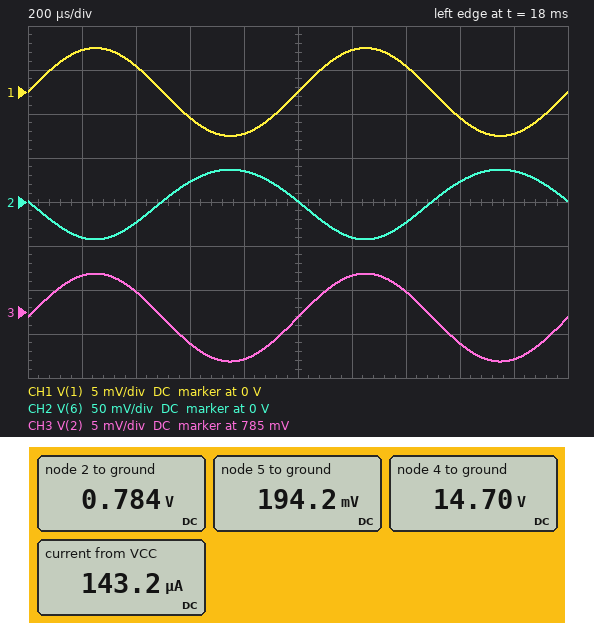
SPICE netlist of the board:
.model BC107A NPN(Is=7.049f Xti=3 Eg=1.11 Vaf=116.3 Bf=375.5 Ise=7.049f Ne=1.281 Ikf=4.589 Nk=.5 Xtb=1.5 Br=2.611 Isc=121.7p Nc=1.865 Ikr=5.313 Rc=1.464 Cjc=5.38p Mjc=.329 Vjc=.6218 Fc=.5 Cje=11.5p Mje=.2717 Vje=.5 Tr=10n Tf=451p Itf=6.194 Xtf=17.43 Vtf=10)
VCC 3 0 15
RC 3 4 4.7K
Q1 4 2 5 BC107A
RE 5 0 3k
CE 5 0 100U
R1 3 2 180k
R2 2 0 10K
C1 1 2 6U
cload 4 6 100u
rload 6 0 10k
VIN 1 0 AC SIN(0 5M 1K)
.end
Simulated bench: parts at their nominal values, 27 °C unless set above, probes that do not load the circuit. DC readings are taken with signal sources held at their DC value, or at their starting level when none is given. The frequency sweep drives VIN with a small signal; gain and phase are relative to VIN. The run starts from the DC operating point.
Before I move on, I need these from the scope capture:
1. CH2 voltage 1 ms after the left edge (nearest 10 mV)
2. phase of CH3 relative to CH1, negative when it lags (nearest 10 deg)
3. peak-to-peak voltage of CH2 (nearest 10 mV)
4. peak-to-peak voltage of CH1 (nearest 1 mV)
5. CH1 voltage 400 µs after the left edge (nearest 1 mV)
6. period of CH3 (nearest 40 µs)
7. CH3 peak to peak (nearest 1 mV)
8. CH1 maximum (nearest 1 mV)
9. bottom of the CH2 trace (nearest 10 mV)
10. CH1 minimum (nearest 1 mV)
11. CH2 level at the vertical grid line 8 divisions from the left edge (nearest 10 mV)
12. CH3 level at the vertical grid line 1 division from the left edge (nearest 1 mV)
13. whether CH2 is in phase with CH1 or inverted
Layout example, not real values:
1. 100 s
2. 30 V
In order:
1. 0 V
2. 0 deg
3. 80 mV
4. 10 mV
5. 3 mV
6. 1.00 ms
7. 10 mV
8. 5 mV
9. -40 mV
10. -5 mV
11. 20 mV
12. 789 mV
13. inverted
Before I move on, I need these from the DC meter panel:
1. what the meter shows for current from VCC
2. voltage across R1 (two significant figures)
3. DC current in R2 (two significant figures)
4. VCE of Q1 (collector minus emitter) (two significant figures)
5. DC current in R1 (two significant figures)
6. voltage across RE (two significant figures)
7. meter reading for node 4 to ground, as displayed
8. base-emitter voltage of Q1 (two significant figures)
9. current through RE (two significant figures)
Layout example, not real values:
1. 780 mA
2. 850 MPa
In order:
1. 143.2 µA
2. 14 V
3. 78 µA
4. 15 V
5. 79 µA
6. 190 mV
7. 14.70 V
8. 590 mV
9. 65 µA
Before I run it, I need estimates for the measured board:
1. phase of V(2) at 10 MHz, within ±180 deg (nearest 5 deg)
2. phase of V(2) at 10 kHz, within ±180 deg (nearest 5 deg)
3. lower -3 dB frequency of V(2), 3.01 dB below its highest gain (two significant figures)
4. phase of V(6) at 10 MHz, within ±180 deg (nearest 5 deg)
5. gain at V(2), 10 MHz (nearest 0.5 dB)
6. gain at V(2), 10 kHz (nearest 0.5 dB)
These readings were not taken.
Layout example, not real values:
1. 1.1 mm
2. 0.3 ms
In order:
1. 0 deg
2. 0 deg
3. 3.2 Hz
4. 155 deg
5. 0 dB
6. 0 dB
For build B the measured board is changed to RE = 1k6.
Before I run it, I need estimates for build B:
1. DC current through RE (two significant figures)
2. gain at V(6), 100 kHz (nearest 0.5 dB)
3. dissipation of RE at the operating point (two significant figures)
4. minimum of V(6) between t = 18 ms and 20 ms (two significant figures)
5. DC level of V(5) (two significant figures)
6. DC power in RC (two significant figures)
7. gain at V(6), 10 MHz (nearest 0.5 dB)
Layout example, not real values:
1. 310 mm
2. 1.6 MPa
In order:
1. 110 µA
2. 22.5 dB
3. 20 µW
4. -72 mV
5. 180 mV
6. 57 µW
7. 22.0 dB
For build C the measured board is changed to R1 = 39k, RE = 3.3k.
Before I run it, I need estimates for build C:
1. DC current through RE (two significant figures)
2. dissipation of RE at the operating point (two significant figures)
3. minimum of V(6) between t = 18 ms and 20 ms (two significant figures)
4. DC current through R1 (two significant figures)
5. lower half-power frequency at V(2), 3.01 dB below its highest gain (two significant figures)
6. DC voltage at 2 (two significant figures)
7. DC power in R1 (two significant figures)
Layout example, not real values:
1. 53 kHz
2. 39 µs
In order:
1. 720 µA
2. 1.7 mW
3. -450 mV
4. 310 µA
5. 3.8 Hz
6. 3.0 V
7. 3.7 mW
